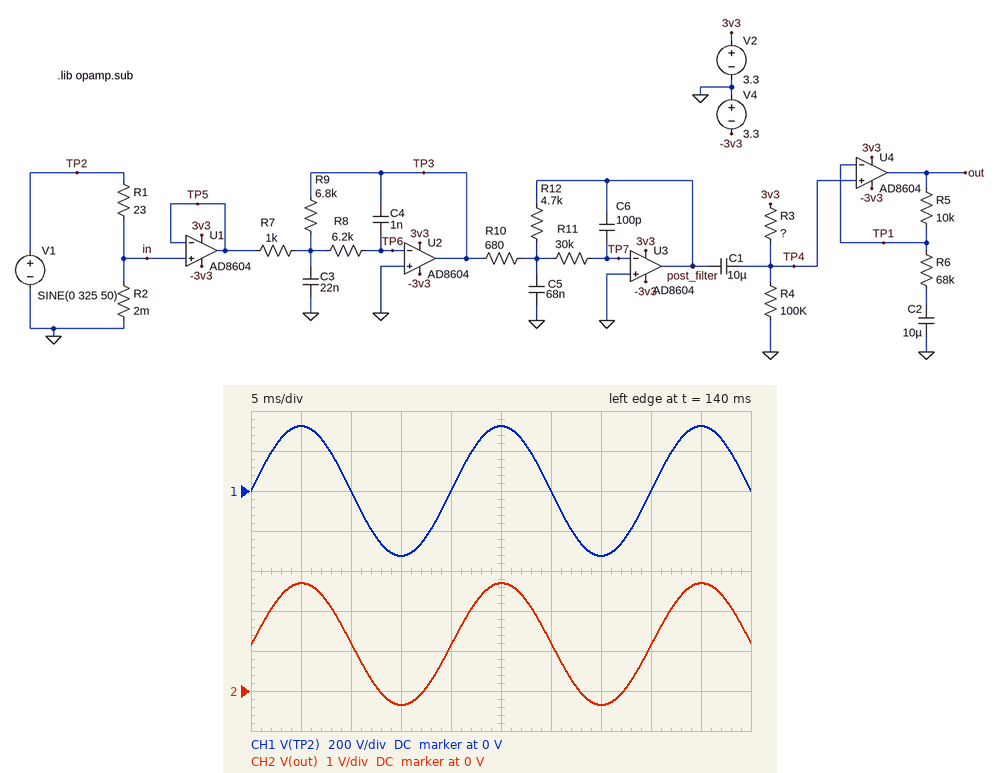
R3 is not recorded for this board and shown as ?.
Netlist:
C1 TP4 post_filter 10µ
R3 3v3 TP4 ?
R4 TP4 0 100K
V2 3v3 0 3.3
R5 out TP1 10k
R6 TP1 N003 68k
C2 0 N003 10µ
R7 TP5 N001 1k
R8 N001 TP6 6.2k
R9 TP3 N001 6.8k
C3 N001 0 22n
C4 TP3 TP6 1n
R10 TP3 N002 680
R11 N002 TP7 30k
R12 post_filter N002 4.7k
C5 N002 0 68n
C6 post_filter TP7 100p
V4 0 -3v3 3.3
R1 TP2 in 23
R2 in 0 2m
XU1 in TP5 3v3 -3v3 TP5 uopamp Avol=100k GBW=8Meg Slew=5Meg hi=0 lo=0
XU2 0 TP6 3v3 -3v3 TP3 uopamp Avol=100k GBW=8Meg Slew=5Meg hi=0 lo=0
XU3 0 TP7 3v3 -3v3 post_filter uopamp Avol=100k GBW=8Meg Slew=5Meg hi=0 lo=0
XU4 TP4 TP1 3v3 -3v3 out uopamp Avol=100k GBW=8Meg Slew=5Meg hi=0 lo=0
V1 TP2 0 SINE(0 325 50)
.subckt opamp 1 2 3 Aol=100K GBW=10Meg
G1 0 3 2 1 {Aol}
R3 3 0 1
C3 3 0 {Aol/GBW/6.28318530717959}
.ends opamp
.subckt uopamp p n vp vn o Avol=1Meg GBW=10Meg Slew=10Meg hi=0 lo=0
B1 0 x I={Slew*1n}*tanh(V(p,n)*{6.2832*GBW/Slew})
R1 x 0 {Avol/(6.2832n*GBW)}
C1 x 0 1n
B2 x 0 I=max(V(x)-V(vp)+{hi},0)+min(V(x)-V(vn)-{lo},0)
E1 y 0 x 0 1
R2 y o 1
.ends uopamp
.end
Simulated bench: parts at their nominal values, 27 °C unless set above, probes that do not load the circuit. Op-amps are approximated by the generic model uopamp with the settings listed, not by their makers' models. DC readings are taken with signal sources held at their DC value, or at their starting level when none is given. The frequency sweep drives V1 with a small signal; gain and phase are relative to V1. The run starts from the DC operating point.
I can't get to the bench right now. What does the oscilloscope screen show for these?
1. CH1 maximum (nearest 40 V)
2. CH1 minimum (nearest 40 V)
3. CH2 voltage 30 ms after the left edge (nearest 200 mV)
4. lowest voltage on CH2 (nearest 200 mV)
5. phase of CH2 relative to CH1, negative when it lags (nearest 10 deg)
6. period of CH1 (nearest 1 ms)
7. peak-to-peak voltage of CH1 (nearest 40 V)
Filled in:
320 V
-320 V
1.2 V
-400 mV
0 deg
20 ms
640 V
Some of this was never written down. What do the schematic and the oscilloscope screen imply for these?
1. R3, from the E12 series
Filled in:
180 kΩ
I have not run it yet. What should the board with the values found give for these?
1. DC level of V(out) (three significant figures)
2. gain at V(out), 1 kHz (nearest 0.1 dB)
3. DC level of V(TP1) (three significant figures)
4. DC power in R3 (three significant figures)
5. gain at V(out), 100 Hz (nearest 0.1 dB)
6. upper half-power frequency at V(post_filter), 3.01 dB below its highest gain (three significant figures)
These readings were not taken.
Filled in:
1.18 V
-46.6 dB
1.18 V
25.0 µW
-46.6 dB
5.13 kHz
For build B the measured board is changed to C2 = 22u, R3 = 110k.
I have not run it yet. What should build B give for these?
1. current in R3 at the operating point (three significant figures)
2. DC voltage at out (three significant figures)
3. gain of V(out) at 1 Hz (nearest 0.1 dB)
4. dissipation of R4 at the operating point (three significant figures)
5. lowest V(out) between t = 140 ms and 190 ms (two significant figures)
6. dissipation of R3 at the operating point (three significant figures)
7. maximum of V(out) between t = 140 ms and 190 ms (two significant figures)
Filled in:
15.7 µA
1.57 V
-47.0 dB
24.7 µW
41 mV
27.2 µW
3.1 V
